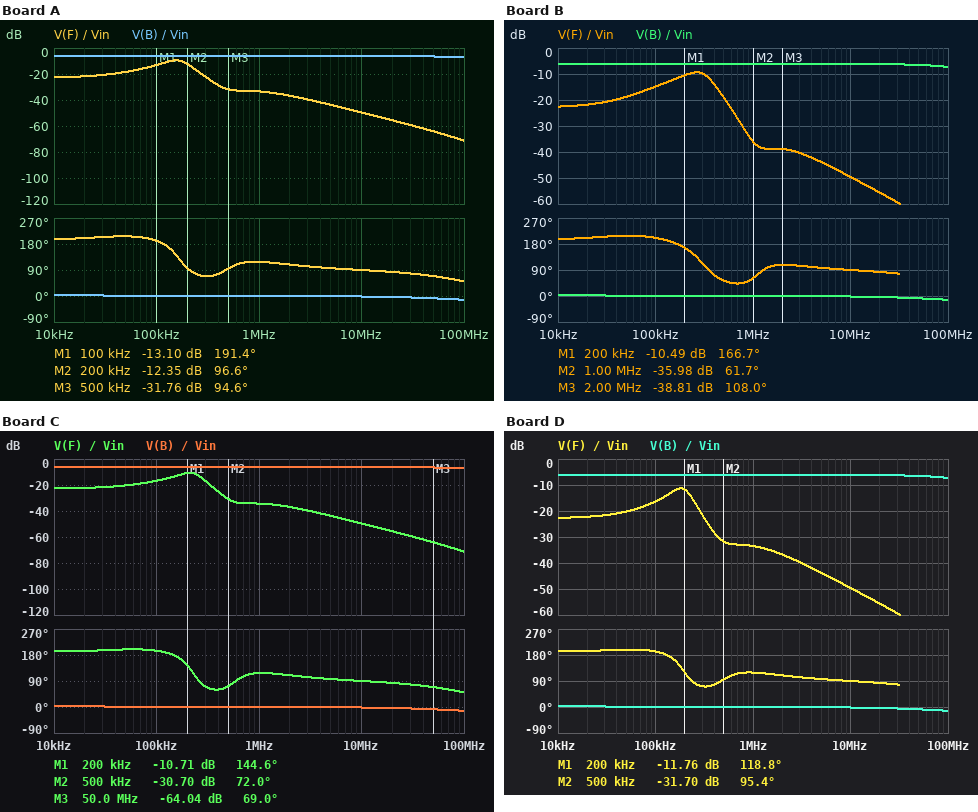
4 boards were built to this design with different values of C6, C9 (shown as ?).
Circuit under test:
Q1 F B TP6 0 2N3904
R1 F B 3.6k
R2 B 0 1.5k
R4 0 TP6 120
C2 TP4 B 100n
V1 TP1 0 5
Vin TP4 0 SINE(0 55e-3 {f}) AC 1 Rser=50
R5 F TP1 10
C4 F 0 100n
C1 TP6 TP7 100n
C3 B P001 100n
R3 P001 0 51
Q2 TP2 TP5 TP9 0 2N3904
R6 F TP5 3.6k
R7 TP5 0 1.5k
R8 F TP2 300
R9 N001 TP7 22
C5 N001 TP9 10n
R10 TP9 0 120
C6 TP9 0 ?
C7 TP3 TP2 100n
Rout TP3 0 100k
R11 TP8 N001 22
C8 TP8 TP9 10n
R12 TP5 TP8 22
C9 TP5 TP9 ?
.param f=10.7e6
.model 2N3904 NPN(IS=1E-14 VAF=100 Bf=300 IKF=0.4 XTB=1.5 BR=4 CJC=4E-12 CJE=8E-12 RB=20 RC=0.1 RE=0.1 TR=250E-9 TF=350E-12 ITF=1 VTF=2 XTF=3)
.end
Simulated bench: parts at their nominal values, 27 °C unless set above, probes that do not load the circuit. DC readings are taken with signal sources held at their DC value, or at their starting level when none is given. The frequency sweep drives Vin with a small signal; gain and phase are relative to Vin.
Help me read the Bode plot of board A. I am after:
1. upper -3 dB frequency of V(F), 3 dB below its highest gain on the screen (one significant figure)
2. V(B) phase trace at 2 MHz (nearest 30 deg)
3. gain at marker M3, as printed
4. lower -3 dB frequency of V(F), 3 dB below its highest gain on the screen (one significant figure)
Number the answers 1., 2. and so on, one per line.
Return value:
1. 200 kHz
2. 0 deg
3. -31.76 dB
4. 100 kHz
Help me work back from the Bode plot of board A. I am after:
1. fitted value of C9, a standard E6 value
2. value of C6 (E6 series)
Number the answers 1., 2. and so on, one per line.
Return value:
1. 33 nF
2. 68 nF
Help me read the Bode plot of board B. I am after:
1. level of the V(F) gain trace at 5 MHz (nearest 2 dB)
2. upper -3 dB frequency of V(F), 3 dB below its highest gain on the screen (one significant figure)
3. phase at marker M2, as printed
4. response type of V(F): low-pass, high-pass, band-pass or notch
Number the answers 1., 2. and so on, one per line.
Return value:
1. -44 dB
2. 400 kHz
3. 61.7 deg
4. band-pass
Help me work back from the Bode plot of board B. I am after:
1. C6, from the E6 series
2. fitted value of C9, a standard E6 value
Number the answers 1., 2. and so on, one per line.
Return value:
1. 68 nF
2. 3.3 nF
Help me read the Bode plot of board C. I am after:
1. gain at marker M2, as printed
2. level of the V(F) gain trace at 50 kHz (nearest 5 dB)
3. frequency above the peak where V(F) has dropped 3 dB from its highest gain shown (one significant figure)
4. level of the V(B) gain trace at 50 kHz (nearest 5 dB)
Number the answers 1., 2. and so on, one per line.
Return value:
1. -30.70 dB
2. -20 dB
3. 300 kHz
4. -5 dB
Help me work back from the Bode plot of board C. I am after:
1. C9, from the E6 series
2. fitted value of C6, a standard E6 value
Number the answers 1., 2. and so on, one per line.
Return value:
1. 22 nF
2. 47 nF
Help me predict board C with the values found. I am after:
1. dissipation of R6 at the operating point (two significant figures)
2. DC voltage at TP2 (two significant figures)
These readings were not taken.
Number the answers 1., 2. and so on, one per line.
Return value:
1. 3.3 mW
2. 3.1 V
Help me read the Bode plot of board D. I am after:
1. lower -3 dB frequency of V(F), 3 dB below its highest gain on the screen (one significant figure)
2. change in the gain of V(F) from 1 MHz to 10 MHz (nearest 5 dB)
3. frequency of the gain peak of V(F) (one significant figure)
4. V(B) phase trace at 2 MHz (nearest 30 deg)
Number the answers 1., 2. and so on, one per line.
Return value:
1. 100 kHz
2. -15 dB
3. 200 kHz
4. 0 deg
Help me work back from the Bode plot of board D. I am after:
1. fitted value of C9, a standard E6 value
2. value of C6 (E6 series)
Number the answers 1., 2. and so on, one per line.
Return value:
1. 33 nF
2. 47 nF
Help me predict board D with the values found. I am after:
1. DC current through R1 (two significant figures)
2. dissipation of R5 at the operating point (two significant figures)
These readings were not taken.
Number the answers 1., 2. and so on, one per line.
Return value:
1. 960 µA
2. 1.9 mW
